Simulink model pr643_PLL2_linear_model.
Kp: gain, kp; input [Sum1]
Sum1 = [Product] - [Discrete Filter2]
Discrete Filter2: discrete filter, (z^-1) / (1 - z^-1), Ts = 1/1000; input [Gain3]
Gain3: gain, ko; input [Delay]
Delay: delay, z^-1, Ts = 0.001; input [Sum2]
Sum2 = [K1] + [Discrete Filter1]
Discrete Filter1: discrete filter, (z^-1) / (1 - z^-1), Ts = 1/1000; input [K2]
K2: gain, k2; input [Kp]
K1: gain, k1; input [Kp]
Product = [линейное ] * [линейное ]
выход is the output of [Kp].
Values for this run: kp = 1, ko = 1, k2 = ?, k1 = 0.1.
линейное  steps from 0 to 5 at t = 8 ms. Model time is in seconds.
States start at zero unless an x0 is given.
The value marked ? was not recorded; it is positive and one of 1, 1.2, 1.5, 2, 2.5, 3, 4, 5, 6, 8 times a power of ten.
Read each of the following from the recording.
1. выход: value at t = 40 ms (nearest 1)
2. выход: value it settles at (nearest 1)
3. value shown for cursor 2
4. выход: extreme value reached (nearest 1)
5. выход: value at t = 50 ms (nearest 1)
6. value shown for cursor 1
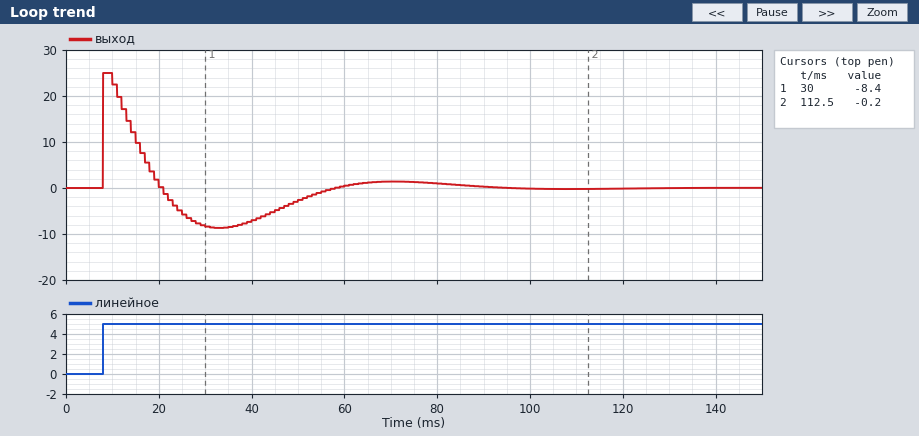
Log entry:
-7
0
-0.2
25
-3
-8.4
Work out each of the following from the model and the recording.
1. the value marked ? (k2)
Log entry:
0.008
